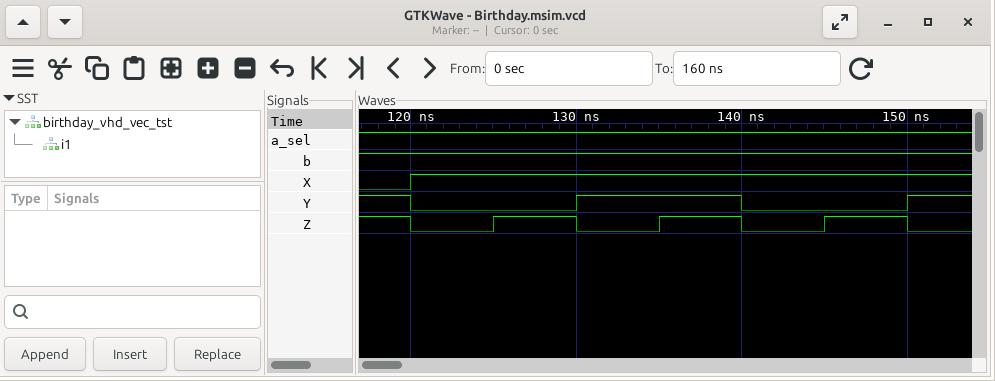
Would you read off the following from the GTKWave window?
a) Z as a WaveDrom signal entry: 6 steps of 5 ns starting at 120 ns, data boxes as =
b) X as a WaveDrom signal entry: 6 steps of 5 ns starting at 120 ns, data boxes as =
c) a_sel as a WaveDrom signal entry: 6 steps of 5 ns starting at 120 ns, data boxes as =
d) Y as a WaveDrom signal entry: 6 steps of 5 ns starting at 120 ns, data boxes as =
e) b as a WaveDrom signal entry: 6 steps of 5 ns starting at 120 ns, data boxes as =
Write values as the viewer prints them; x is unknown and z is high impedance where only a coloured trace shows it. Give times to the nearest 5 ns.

{name: 'Z', wave: '010101'}
{name: 'X', wave: '1.....'}
{name: 'a_sel', wave: '1.....'}
{name: 'Y', wave: '0.1.0.'}
{name: 'b', wave: '1.....'}
